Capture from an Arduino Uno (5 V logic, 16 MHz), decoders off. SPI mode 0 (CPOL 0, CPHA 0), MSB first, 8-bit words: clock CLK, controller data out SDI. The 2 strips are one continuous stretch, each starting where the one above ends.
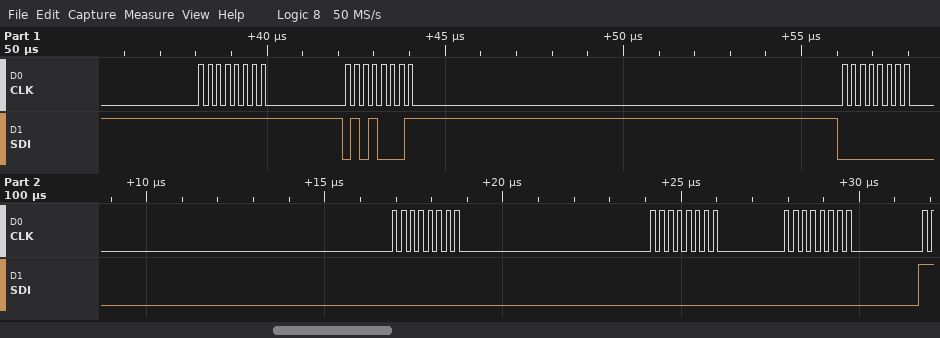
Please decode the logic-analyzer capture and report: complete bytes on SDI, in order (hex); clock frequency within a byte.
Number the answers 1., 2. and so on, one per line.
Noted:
1. FF 51 00 00 00 00
2. 4 MHz
